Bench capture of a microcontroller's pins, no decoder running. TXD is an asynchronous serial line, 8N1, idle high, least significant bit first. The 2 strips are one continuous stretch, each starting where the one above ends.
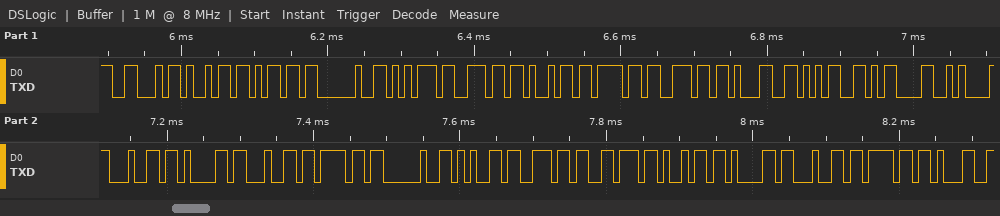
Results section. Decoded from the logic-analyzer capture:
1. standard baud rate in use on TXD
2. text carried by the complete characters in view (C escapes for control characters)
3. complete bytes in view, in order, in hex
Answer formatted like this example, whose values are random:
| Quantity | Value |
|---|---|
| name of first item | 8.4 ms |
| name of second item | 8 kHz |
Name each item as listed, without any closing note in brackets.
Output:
| Quantity | Value |
|---|---|
| standard baud rate in use on TXD | 115200 baud |
| text carried by the complete characters in view | "Fim union15\r\ndado enviado1" |
| complete bytes in view, in order, in hex | 46 69 6D 20 75 6E 69 6F 6E 31 35 0D 0A 64 61 64 6F 20 65 6E 76 69 61 64 6F 31 |
